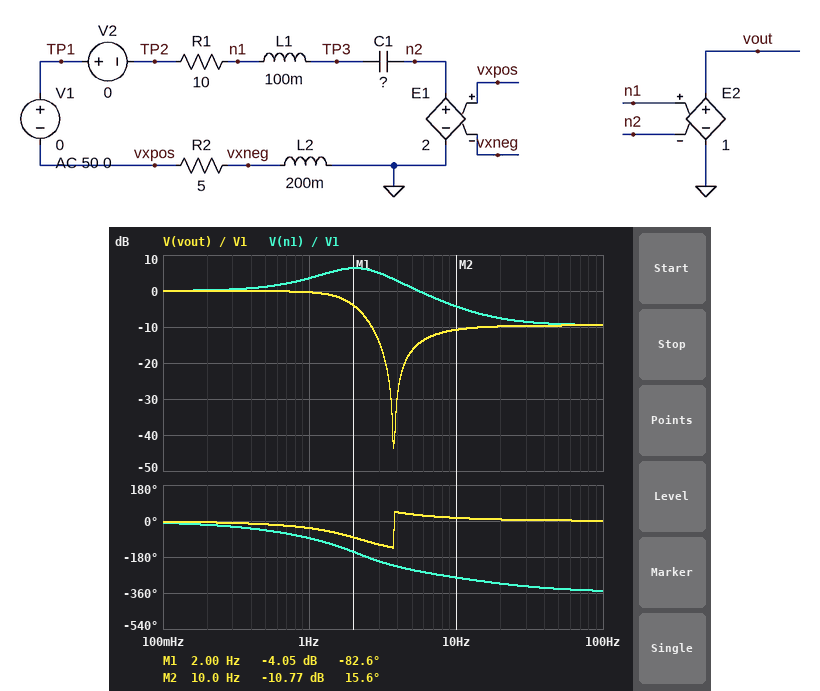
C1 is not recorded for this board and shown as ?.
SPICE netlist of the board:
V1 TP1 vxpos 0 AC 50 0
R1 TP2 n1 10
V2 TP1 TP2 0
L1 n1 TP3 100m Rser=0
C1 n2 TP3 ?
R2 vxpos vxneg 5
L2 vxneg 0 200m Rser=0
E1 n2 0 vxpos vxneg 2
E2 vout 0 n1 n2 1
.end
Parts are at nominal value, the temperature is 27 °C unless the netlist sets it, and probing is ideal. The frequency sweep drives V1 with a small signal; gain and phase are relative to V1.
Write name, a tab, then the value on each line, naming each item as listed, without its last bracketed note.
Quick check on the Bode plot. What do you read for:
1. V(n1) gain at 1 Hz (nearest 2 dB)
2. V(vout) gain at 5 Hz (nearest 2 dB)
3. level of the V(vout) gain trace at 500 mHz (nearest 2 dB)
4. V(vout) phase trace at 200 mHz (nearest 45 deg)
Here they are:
V(n1) gain at 1 Hz	4 dB
V(vout) gain at 5 Hz	-16 dB
level of the V(vout) gain trace at 500 mHz	0 dB
V(vout) phase trace at 200 mHz	0 deg
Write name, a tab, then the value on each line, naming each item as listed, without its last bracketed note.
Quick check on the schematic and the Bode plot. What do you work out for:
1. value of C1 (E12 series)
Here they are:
value of C1	18 mF
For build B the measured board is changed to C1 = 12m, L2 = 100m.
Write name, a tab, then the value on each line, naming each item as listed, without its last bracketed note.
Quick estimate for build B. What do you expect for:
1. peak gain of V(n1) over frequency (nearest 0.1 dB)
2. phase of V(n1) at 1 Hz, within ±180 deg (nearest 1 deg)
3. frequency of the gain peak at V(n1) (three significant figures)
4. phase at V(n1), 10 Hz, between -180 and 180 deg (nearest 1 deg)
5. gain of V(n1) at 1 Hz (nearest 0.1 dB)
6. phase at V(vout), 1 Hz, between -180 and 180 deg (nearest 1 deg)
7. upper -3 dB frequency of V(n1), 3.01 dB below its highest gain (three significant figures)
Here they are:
peak gain of V(n1) over frequency	6.2 dB
phase of V(n1) at 1 Hz, within ±180 deg	-61 deg
frequency of the gain peak at V(n1)	3.08 Hz
phase at V(n1), 10 Hz, between -180 and 180 deg	88 deg
gain of V(n1) at 1 Hz	1.9 dB
phase at V(vout), 1 Hz, between -180 and 180 deg	-23 deg
upper -3 dB frequency of V(n1), 3.01 dB below its highest gain	5.70 Hz
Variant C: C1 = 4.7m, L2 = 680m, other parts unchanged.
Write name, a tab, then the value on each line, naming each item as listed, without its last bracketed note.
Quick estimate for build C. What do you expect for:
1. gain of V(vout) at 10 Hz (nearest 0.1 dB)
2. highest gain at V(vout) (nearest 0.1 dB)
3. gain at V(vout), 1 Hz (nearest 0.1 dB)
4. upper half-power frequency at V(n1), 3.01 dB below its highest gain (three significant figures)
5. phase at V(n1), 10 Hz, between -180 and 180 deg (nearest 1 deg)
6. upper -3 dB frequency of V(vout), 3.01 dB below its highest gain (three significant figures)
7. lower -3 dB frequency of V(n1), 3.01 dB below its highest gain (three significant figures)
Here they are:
gain of V(vout) at 10 Hz	-24.0 dB
highest gain at V(vout)	7.3 dB
gain at V(vout), 1 Hz	1.1 dB
upper half-power frequency at V(n1), 3.01 dB below its highest gain	3.05 Hz
phase at V(n1), 10 Hz, between -180 and 180 deg	80 deg
upper -3 dB frequency of V(vout), 3.01 dB below its highest gain	2.96 Hz
lower -3 dB frequency of V(n1), 3.01 dB below its highest gain	2.01 Hz
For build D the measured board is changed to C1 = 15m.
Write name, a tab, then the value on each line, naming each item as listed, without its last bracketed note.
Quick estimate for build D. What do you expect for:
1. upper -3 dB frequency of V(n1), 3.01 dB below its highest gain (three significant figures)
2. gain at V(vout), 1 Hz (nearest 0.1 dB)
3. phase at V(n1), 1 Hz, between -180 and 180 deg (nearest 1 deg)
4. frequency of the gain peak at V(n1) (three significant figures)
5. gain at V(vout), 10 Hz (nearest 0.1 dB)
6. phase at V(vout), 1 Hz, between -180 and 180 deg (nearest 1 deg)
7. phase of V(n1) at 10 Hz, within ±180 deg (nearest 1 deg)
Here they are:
upper -3 dB frequency of V(n1), 3.01 dB below its highest gain	3.86 Hz
gain at V(vout), 1 Hz	-0.1 dB
phase at V(n1), 1 Hz, between -180 and 180 deg	-75 deg
frequency of the gain peak at V(n1)	2.24 Hz
gain at V(vout), 10 Hz	-11.0 dB
phase at V(vout), 1 Hz, between -180 and 180 deg	-30 deg
phase of V(n1) at 10 Hz, within ±180 deg	78 deg
